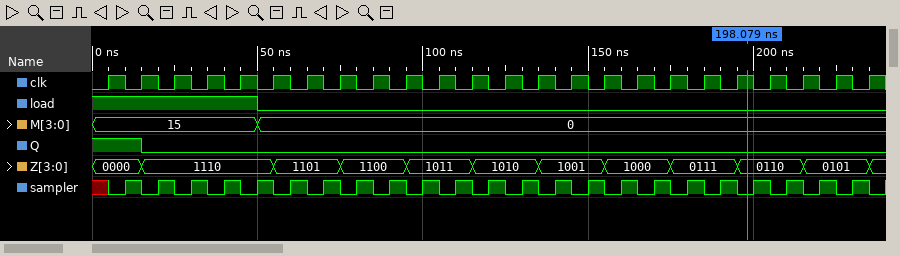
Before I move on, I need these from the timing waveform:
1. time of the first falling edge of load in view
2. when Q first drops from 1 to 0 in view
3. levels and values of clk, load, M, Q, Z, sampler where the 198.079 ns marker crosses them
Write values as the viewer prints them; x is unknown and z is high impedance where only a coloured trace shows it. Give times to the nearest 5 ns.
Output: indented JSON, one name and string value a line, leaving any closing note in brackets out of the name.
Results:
{
  "time of the first falling edge of load in view": "50 ns",
  "when Q first drops from 1 to 0 in view": "15 ns",
  "levels and values of clk, load, M, Q, Z, sampler where the 198.079 ns marker crosses them": "clk=1, load=0, M=0, Q=0, Z=0110, sampler=0"
}
